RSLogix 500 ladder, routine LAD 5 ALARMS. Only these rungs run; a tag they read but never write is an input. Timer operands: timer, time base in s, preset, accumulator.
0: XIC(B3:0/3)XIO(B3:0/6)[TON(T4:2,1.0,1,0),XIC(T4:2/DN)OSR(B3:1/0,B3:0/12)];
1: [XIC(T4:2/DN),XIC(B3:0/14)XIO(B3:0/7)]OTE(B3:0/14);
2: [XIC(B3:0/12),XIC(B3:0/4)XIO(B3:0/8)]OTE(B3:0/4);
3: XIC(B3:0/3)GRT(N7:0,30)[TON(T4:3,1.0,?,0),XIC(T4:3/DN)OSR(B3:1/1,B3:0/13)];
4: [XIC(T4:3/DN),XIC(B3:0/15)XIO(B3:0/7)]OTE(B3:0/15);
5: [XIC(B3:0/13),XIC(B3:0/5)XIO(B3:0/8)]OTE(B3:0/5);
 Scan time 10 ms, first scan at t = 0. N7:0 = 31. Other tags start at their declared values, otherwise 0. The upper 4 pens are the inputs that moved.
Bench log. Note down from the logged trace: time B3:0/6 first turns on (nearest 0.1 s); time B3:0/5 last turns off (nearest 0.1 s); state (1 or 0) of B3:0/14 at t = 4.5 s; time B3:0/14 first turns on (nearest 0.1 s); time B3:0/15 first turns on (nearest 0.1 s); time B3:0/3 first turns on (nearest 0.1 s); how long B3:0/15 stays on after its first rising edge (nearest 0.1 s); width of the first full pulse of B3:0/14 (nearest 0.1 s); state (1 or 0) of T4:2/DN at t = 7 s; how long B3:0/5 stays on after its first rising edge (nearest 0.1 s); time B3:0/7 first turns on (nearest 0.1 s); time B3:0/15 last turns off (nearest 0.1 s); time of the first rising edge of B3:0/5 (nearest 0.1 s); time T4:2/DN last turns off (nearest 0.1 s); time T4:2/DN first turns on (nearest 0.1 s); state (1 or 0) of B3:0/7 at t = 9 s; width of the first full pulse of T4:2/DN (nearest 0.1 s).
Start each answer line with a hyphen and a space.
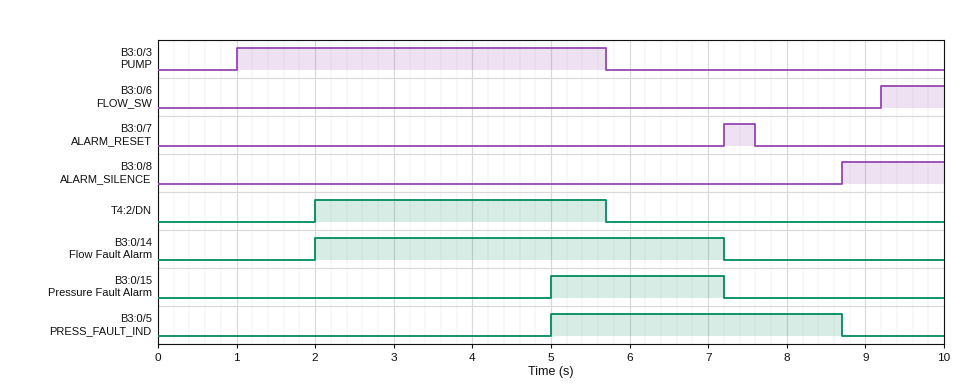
- 9.2 s
- 8.7 s
- 1
- 2.0 s
- 5.0 s
- 1.0 s
- 2.2 s
- 5.2 s
- 0
- 3.7 s
- 7.2 s
- 7.2 s
- 5.0 s
- 5.7 s
- 2.0 s
- 0
- 3.7 s
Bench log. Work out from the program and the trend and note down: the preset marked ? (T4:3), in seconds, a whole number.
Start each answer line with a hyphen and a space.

- 4 s
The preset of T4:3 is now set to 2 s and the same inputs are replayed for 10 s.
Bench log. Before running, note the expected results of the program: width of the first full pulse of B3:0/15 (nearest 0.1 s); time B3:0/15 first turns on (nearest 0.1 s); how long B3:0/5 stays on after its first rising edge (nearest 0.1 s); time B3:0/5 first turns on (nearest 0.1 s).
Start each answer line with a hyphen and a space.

- 4.2 s
- 3.0 s
- 5.7 s
- 3.0 s
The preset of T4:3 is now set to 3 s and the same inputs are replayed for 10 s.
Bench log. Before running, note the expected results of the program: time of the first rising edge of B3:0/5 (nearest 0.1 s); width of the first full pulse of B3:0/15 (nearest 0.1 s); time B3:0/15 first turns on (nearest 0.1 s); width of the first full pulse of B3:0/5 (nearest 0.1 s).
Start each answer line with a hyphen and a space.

- 4.0 s
- 3.2 s
- 4.0 s
- 4.7 s
